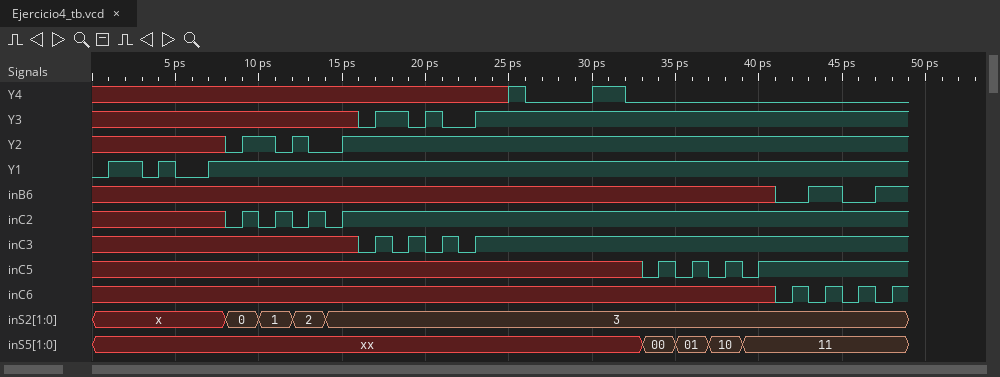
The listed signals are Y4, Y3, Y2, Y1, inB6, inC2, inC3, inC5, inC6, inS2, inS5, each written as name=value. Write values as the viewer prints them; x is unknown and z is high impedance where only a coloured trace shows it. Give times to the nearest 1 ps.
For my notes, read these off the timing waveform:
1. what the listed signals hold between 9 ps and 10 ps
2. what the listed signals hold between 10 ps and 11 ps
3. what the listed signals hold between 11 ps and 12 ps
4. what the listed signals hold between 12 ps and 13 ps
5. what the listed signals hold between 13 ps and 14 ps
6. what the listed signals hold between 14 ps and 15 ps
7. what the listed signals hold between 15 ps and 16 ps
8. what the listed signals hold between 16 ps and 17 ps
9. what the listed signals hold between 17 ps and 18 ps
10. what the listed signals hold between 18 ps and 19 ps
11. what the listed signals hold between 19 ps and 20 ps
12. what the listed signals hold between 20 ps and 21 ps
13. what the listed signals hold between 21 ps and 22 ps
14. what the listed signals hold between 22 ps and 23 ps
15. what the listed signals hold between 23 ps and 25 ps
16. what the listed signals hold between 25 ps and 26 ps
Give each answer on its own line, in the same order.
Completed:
Y4=x, Y3=x, Y2=1, Y1=1, inB6=x, inC2=1, inC3=x, inC5=x, inC6=x, inS2=0, inS5=xx
Y4=x, Y3=x, Y2=1, Y1=1, inB6=x, inC2=0, inC3=x, inC5=x, inC6=x, inS2=1, inS5=xx
Y4=x, Y3=x, Y2=0, Y1=1, inB6=x, inC2=1, inC3=x, inC5=x, inC6=x, inS2=1, inS5=xx
Y4=x, Y3=x, Y2=1, Y1=1, inB6=x, inC2=0, inC3=x, inC5=x, inC6=x, inS2=2, inS5=xx
Y4=x, Y3=x, Y2=0, Y1=1, inB6=x, inC2=1, inC3=x, inC5=x, inC6=x, inS2=2, inS5=xx
Y4=x, Y3=x, Y2=0, Y1=1, inB6=x, inC2=0, inC3=x, inC5=x, inC6=x, inS2=3, inS5=xx
Y4=x, Y3=x, Y2=1, Y1=1, inB6=x, inC2=1, inC3=x, inC5=x, inC6=x, inS2=3, inS5=xx
Y4=x, Y3=0, Y2=1, Y1=1, inB6=x, inC2=1, inC3=0, inC5=x, inC6=x, inS2=3, inS5=xx
Y4=x, Y3=1, Y2=1, Y1=1, inB6=x, inC2=1, inC3=1, inC5=x, inC6=x, inS2=3, inS5=xx
Y4=x, Y3=1, Y2=1, Y1=1, inB6=x, inC2=1, inC3=0, inC5=x, inC6=x, inS2=3, inS5=xx
Y4=x, Y3=0, Y2=1, Y1=1, inB6=x, inC2=1, inC3=1, inC5=x, inC6=x, inS2=3, inS5=xx
Y4=x, Y3=1, Y2=1, Y1=1, inB6=x, inC2=1, inC3=0, inC5=x, inC6=x, inS2=3, inS5=xx
Y4=x, Y3=0, Y2=1, Y1=1, inB6=x, inC2=1, inC3=1, inC5=x, inC6=x, inS2=3, inS5=xx
Y4=x, Y3=0, Y2=1, Y1=1, inB6=x, inC2=1, inC3=0, inC5=x, inC6=x, inS2=3, inS5=xx
Y4=x, Y3=1, Y2=1, Y1=1, inB6=x, inC2=1, inC3=1, inC5=x, inC6=x, inS2=3, inS5=xx
Y4=1, Y3=1, Y2=1, Y1=1, inB6=x, inC2=1, inC3=1, inC5=x, inC6=x, inS2=3, inS5=xx
